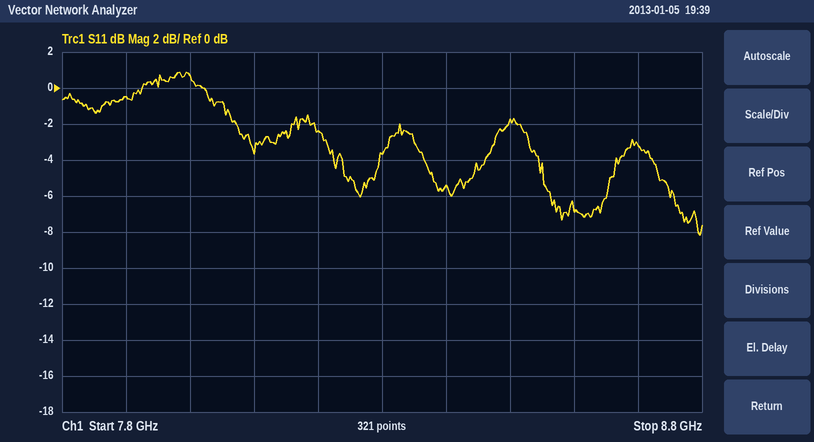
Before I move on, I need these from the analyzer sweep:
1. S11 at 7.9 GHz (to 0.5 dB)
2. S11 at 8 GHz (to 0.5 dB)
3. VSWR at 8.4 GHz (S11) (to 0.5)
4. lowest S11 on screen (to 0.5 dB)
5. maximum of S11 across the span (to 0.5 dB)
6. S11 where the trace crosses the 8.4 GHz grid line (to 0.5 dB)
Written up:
-0.5 dB
0.5 dB
3.5
-8.0 dB
1.0 dB
-5.5 dB
